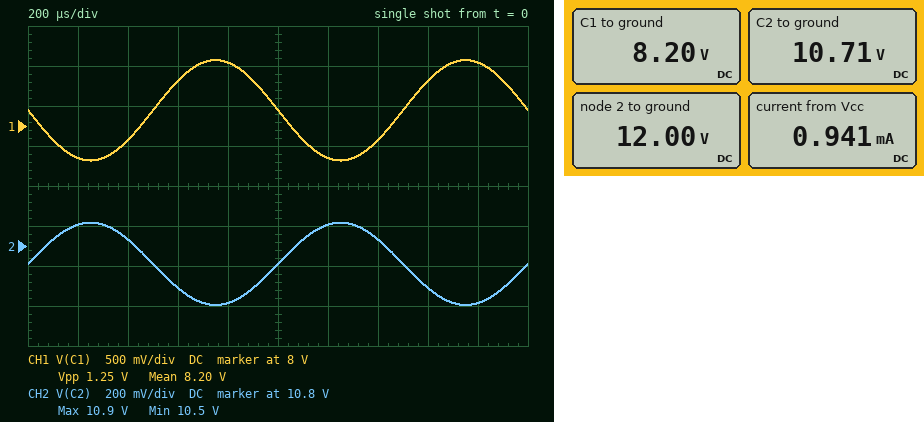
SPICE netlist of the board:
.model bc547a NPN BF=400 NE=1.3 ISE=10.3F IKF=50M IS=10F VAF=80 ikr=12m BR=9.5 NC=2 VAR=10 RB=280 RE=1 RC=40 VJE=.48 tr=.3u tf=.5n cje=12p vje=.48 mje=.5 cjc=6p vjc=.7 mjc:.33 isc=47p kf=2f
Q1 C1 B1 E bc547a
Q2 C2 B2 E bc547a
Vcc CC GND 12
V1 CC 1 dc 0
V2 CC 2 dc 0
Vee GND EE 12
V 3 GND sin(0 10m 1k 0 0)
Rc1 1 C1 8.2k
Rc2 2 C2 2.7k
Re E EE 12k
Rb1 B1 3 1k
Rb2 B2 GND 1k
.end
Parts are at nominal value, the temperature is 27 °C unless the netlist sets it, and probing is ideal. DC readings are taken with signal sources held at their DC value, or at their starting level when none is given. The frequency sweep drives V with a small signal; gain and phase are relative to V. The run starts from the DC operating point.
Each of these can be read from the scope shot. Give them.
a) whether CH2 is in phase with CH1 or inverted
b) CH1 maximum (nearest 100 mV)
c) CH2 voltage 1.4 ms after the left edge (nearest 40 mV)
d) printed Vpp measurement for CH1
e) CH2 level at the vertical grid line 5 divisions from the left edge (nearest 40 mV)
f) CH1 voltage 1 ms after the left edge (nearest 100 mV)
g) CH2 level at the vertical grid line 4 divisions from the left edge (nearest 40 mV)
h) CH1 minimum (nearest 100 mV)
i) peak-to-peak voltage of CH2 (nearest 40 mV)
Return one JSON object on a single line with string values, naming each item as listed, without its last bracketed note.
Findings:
{"whether CH2 is in phase with CH1 or inverted": "inverted", "CH1 maximum": "8.8 V", "CH2 voltage 1.4 ms after the left edge": "10.84 V", "printed Vpp measurement for CH1": "1.25 V", "CH2 level at the vertical grid line 5 divisions from the left edge": "10.72 V", "CH1 voltage 1 ms after the left edge": "8.2 V", "CH2 level at the vertical grid line 4 divisions from the left edge": "10.52 V", "CH1 minimum": "7.6 V", "peak-to-peak voltage of CH2": "400 mV"}
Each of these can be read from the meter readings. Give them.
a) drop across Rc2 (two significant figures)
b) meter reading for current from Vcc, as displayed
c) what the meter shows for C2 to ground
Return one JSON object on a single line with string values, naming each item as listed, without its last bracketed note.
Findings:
{"drop across Rc2": "1.3 V", "meter reading for current from Vcc, as displayed": "0.941 mA", "what the meter shows for C2 to ground": "10.71 V"}
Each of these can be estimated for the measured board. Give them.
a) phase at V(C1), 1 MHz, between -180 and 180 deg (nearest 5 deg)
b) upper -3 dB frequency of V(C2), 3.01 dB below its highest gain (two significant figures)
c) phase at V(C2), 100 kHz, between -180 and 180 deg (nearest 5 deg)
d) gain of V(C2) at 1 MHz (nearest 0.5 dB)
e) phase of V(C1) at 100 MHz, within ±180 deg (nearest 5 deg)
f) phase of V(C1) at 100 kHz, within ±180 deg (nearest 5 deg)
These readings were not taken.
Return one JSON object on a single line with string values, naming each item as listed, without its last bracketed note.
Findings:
{"phase at V(C1), 1 MHz, between -180 and 180 deg": "115 deg", "upper -3 dB frequency of V(C2), 3.01 dB below its highest gain": "470 kHz", "phase at V(C2), 100 kHz, between -180 and 180 deg": "-10 deg", "gain of V(C2) at 1 MHz": "19.0 dB", "phase of V(C1) at 100 MHz, within ±180 deg": "10 deg", "phase of V(C1) at 100 kHz, within ±180 deg": "170 deg"}
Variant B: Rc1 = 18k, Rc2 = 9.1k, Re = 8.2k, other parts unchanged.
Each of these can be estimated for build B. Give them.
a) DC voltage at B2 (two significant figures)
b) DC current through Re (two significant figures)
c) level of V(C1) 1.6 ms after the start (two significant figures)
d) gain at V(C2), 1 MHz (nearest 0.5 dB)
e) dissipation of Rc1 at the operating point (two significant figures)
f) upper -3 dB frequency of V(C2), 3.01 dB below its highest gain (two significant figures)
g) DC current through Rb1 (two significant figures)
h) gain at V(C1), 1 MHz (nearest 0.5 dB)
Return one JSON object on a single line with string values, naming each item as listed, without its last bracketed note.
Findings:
{"DC voltage at B2": "-4.1 mV", "DC current through Re": "1.4 mA", "level of V(C1) 1.6 ms after the start": "1.1 V", "gain at V(C2), 1 MHz": "19.0 dB", "dissipation of Rc1 at the operating point": "7.9 mW", "upper -3 dB frequency of V(C2), 3.01 dB below its highest gain": "89 kHz", "DC current through Rb1": "4.1 µA", "gain at V(C1), 1 MHz": "23.5 dB"}
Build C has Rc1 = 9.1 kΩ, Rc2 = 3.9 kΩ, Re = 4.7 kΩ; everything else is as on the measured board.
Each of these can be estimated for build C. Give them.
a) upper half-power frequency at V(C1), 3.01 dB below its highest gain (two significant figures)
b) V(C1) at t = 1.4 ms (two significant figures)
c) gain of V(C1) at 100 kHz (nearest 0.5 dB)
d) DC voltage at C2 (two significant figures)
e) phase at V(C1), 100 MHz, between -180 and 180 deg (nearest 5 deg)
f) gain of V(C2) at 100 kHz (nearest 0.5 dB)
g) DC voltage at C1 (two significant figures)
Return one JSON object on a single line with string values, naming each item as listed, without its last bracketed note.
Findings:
{"upper half-power frequency at V(C1), 3.01 dB below its highest gain": "150 kHz", "V(C1) at t = 1.4 ms": "640 mV", "gain of V(C1) at 100 kHz": "41.5 dB", "DC voltage at C2": "7.2 V", "phase at V(C1), 100 MHz, between -180 and 180 deg": "15 deg", "gain of V(C2) at 100 kHz": "34.0 dB", "DC voltage at C1": "1.5 V"}
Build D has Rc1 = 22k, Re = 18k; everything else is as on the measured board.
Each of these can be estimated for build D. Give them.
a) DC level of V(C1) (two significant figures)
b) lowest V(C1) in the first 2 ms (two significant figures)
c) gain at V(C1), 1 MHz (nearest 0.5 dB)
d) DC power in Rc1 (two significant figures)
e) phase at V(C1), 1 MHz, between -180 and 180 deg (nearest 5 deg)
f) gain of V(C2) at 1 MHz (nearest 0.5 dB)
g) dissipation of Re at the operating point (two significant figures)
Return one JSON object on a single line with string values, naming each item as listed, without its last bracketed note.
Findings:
{"DC level of V(C1)": "5.3 V", "lowest V(C1) in the first 2 ms": "4.2 V", "gain at V(C1), 1 MHz": "29.5 dB", "DC power in Rc1": "2.0 mW", "phase at V(C1), 1 MHz, between -180 and 180 deg": "100 deg", "gain of V(C2) at 1 MHz": "12.0 dB", "dissipation of Re at the operating point": "7.2 mW"}
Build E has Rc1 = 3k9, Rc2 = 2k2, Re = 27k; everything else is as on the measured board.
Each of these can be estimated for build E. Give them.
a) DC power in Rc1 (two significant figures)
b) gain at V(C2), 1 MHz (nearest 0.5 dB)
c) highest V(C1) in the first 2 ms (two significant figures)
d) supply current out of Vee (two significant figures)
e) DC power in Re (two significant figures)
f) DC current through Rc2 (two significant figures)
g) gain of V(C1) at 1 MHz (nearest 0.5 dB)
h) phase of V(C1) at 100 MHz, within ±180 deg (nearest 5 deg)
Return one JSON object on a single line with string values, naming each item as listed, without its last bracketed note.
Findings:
{"DC power in Rc1": "170 µW", "gain at V(C2), 1 MHz": "16.5 dB", "highest V(C1) in the first 2 ms": "11 V", "supply current out of Vee": "420 µA", "DC power in Re": "4.8 mW", "DC current through Rc2": "210 µA", "gain of V(C1) at 1 MHz": "21.5 dB", "phase of V(C1) at 100 MHz, within ±180 deg": "10 deg"}
